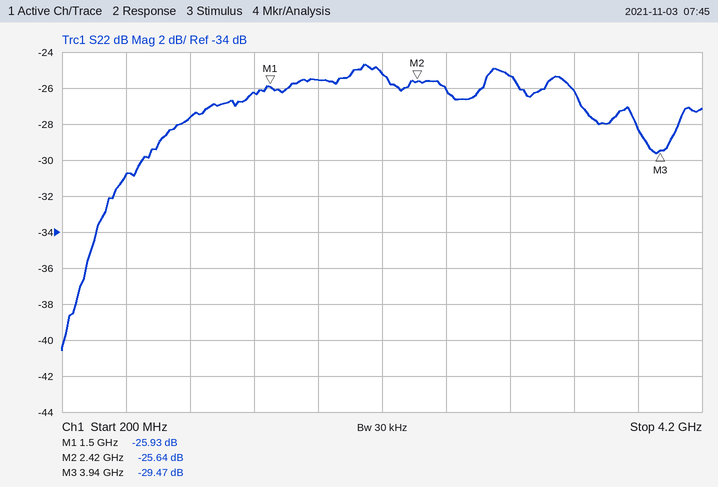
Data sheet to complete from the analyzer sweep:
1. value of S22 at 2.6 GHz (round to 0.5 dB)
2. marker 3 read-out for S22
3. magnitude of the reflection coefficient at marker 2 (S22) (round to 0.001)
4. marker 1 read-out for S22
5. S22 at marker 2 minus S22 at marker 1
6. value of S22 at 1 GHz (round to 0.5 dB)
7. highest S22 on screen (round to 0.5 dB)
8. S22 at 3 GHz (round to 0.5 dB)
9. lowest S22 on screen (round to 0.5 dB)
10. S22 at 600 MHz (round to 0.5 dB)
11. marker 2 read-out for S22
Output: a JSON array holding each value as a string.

["-26.0 dB", "-29.47 dB", "0.052", "-25.93 dB", "0.29 dB", "-27.5 dB", "-24.5 dB", "-25.5 dB", "-40.5 dB", "-31.0 dB", "-25.64 dB"]
